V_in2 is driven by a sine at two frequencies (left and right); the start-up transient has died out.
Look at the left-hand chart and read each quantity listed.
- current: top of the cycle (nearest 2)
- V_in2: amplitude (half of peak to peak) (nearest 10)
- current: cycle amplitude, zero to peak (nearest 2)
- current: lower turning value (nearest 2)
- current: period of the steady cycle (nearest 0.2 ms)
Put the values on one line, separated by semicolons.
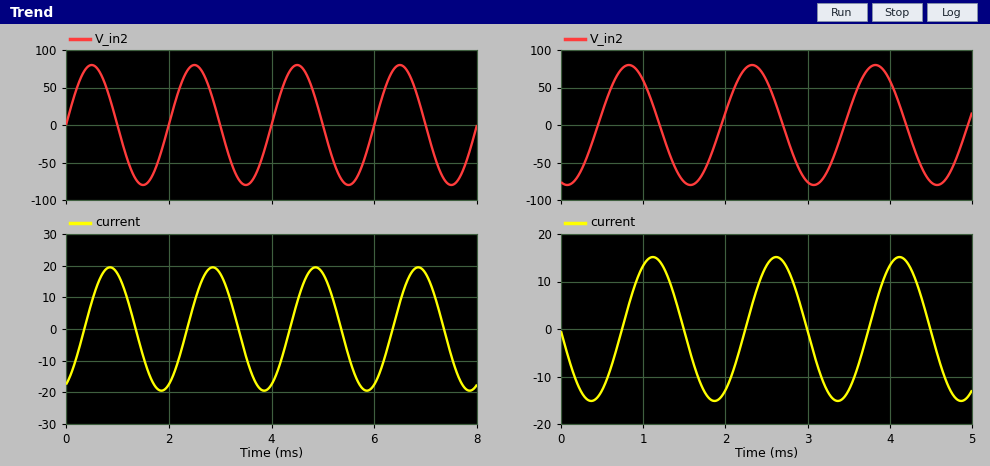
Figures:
20; 80; 20; -20; 2.0 ms
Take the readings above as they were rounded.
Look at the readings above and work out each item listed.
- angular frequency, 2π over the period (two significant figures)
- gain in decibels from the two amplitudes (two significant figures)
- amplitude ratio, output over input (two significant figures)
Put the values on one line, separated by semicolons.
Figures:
3.1 rad/ms; -12 dB; 0.25
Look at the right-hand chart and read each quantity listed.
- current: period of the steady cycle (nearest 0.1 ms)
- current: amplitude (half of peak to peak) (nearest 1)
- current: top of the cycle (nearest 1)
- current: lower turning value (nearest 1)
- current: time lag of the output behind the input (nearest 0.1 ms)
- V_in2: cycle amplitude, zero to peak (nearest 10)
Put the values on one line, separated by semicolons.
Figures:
1.5 ms; 15; 15; -15; 0.3 ms; 80
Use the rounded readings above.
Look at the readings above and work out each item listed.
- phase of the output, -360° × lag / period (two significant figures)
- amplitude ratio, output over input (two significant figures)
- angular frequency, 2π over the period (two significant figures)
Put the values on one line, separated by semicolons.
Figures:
-72°; 0.19; 4.2 rad/ms
